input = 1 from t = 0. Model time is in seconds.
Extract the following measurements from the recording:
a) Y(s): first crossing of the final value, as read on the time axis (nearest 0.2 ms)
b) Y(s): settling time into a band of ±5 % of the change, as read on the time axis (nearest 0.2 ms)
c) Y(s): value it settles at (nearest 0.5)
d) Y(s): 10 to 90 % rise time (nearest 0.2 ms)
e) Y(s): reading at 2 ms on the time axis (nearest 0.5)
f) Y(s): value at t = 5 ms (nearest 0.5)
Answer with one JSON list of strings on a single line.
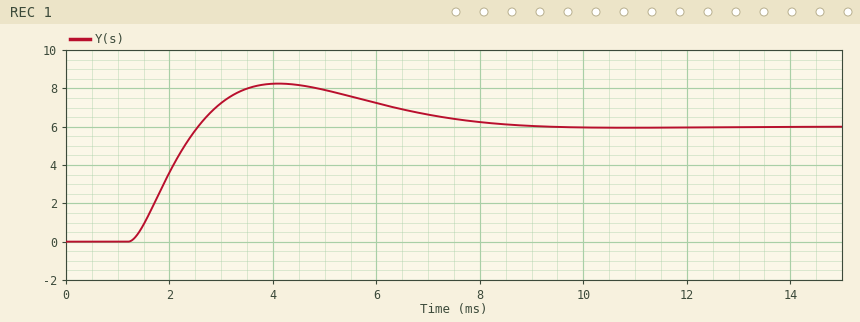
["2.6 ms", "7.8 ms", "6.0", "1.0 ms", "3.5", "8.0"]
